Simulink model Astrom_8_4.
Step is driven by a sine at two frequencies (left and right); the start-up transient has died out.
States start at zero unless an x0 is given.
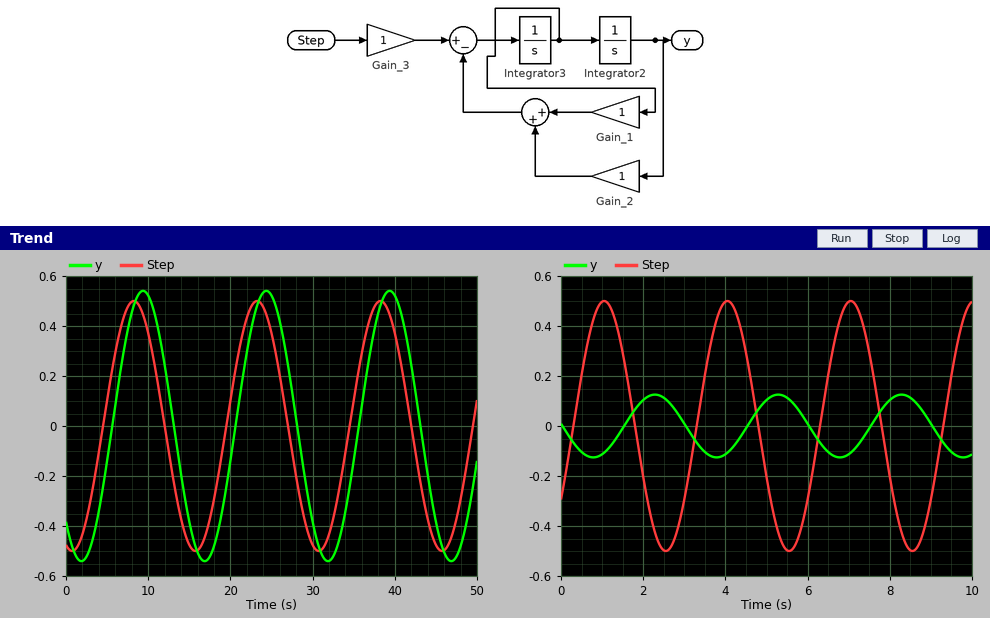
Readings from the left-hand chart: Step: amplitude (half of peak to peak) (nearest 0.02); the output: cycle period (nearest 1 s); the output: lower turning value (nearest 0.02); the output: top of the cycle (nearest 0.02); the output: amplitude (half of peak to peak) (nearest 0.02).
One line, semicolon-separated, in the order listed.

0.50; 15 s; -0.54; 0.54; 0.54
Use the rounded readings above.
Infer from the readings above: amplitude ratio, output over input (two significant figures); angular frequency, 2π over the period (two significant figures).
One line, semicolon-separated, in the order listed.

1.1; 0.42 rad/s
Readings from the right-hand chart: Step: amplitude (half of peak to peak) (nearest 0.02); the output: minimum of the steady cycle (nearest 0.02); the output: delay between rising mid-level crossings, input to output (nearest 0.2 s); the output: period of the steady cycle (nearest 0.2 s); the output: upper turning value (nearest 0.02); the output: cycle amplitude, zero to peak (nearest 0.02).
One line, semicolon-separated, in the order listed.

0.50; -0.12; 1.2 s; 3.0 s; 0.12; 0.12
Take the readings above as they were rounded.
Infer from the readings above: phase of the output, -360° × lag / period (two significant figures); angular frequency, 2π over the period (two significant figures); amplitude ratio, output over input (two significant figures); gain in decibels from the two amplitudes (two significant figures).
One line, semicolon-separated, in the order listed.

-140°; 2.1 rad/s; 0.24; -12 dB
